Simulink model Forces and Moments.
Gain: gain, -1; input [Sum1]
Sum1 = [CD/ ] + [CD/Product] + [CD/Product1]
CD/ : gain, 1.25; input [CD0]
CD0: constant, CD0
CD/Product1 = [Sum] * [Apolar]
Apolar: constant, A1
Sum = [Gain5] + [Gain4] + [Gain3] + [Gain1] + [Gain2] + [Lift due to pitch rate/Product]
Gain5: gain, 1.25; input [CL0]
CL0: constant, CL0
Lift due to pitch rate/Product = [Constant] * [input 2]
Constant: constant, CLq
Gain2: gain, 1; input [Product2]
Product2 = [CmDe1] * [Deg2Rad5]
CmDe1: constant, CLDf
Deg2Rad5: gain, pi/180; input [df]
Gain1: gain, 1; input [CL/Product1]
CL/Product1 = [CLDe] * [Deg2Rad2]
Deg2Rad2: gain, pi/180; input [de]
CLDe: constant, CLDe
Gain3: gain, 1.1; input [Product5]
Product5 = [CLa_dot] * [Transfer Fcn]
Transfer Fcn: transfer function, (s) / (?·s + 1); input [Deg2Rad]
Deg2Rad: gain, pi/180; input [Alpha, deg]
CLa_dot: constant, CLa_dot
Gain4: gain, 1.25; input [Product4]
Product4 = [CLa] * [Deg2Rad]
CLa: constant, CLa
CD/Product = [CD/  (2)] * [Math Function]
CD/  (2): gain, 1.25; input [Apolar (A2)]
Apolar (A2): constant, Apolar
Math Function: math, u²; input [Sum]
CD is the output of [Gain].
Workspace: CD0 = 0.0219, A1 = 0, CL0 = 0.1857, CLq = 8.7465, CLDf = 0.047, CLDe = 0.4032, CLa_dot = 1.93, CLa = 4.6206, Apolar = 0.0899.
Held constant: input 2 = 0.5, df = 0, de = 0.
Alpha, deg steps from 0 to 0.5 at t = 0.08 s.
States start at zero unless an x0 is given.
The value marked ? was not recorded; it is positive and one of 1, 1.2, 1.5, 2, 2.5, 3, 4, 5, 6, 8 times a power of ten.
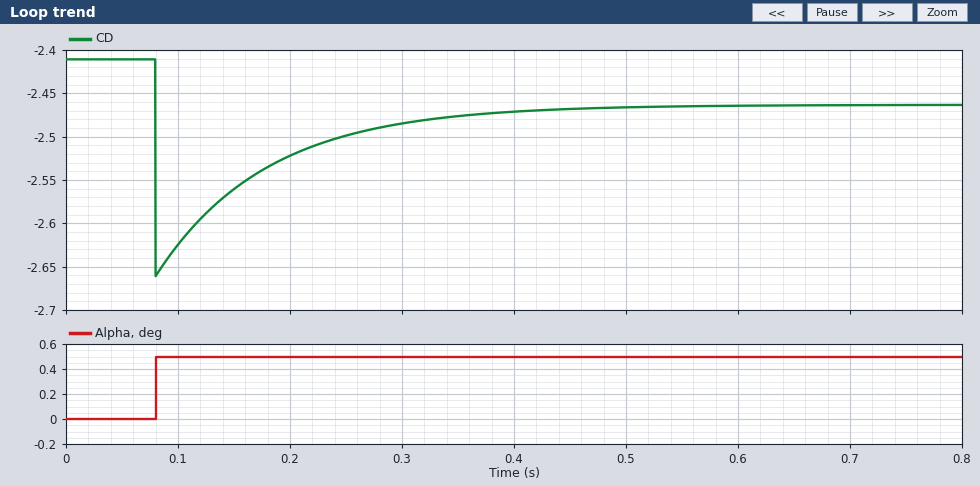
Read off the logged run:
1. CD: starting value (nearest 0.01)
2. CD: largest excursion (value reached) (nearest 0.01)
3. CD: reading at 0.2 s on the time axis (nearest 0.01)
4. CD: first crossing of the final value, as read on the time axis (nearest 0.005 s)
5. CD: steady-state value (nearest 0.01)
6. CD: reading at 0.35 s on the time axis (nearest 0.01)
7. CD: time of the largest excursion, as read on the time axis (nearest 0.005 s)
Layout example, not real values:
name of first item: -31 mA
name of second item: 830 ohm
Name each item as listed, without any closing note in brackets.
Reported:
CD: starting value: -2.41
CD: largest excursion (value reached): -2.66
CD: reading at 0.2 s on the time axis: -2.52
CD: first crossing of the final value, as read on the time axis: 0.080 s
CD: steady-state value: -2.46
CD: reading at 0.35 s on the time axis: -2.48
CD: time of the largest excursion, as read on the time axis: 0.080 s
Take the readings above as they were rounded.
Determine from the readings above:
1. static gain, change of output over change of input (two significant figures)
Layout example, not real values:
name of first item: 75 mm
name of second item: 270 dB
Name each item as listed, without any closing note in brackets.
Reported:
static gain, change of output over change of input: -0.100
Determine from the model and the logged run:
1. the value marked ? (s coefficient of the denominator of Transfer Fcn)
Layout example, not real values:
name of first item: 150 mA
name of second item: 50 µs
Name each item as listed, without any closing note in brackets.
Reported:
the value marked ?: 0.1
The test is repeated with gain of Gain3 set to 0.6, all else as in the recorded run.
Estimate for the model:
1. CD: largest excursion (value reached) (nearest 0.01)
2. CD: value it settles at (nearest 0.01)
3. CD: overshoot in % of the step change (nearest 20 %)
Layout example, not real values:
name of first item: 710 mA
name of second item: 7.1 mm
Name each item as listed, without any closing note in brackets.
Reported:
CD: largest excursion (value reached): -2.57
CD: value it settles at: -2.46
CD: overshoot in % of the step change: 200 %
